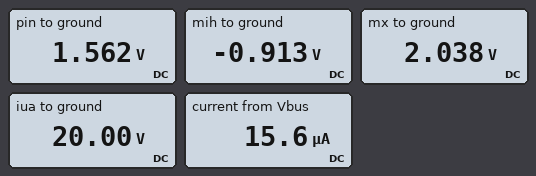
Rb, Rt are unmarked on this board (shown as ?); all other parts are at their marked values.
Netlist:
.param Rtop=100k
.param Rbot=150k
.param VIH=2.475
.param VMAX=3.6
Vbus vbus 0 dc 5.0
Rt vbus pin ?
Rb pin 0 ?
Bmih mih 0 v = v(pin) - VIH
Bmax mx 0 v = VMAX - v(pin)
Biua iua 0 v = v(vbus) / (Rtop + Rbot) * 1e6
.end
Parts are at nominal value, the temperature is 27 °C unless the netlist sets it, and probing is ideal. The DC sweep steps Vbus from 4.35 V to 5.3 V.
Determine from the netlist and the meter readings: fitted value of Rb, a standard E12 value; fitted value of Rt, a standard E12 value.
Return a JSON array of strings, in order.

["100 kΩ", "220 kΩ"]
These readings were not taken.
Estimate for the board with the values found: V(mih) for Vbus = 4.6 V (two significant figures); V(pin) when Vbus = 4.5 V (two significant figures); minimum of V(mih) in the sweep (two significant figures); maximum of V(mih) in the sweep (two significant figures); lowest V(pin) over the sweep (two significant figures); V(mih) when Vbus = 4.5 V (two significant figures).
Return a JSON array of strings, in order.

["-1.0 V", "1.4 V", "-1.1 V", "-820 mV", "1.4 V", "-1.1 V"]
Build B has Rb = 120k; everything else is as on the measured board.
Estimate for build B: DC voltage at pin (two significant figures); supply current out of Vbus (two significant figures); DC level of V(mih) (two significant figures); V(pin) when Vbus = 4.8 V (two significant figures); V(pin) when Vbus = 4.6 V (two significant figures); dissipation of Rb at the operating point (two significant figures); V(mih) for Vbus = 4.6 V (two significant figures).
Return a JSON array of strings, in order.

["1.8 V", "15 µA", "-710 mV", "1.7 V", "1.6 V", "26 µW", "-850 mV"]
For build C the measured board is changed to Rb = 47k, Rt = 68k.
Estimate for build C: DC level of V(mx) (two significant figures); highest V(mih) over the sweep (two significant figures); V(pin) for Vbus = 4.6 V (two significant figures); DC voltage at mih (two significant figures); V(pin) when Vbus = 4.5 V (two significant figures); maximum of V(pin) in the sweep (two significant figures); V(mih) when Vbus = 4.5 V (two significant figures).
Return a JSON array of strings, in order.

["1.6 V", "-310 mV", "1.9 V", "-430 mV", "1.8 V", "2.2 V", "-640 mV"]
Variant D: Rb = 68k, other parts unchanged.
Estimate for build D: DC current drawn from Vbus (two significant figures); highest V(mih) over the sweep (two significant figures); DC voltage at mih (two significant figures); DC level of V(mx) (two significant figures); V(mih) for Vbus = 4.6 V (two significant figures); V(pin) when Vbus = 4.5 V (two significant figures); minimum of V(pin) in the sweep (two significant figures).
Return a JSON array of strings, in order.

["17 µA", "-1.2 V", "-1.3 V", "2.4 V", "-1.4 V", "1.1 V", "1.0 V"]
